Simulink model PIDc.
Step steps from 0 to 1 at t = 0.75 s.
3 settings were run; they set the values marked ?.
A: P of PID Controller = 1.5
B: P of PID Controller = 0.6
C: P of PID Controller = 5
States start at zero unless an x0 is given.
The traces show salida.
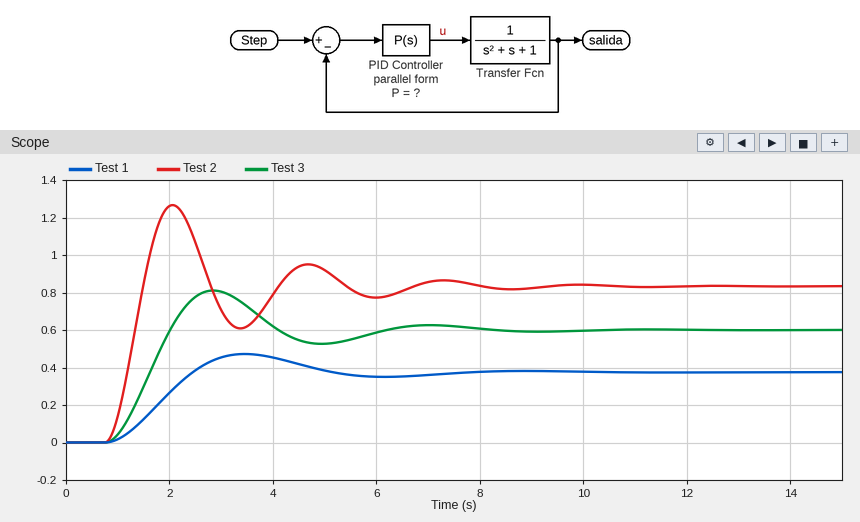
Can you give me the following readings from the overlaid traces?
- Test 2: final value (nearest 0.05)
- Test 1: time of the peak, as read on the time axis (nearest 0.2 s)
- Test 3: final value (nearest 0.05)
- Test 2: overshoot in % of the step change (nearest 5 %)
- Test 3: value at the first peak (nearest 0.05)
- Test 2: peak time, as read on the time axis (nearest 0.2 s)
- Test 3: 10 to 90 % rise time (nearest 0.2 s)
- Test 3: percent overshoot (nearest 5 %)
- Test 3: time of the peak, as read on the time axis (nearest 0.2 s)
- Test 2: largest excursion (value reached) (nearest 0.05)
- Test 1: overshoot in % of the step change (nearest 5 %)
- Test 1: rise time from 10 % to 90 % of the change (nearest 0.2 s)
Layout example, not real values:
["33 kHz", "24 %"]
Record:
["0.85", "3.4 s", "0.60", "50 %", "0.80", "2.0 s", "0.8 s", "35 %", "2.8 s", "1.25", "25 %", "1.2 s"]
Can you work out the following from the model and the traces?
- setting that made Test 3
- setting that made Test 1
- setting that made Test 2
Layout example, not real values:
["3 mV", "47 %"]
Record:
["A", "B", "C"]
